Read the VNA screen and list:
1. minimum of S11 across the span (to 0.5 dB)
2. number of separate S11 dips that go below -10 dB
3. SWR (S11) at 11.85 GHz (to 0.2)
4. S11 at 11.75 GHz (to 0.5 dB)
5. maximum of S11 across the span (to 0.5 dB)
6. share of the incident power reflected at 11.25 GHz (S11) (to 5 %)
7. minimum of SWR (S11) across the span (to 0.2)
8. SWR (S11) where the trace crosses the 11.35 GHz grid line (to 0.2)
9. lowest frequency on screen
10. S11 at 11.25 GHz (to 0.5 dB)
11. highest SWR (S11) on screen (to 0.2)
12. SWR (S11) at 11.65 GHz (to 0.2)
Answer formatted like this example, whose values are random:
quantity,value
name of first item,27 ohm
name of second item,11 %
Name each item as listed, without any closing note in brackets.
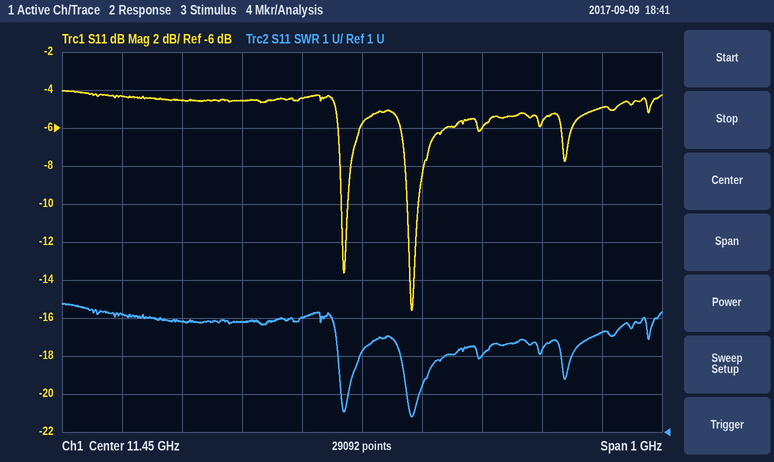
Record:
quantity,value
minimum of S11 across the span,-15.5 dB
number of separate S11 dips that go below -10 dB,2
SWR (S11) at 11.85 GHz,3.6
S11 at 11.75 GHz,-5.5 dB
maximum of S11 across the span,-4.0 dB
share of the incident power reflected at 11.25 GHz (S11),35 %
minimum of SWR (S11) across the span,1.4
SWR (S11) where the trace crosses the 11.35 GHz grid line,4.0
lowest frequency on screen,10.95 GHz
S11 at 11.25 GHz,-4.5 dB
highest SWR (S11) on screen,4.4
SWR (S11) at 11.65 GHz,3.0
